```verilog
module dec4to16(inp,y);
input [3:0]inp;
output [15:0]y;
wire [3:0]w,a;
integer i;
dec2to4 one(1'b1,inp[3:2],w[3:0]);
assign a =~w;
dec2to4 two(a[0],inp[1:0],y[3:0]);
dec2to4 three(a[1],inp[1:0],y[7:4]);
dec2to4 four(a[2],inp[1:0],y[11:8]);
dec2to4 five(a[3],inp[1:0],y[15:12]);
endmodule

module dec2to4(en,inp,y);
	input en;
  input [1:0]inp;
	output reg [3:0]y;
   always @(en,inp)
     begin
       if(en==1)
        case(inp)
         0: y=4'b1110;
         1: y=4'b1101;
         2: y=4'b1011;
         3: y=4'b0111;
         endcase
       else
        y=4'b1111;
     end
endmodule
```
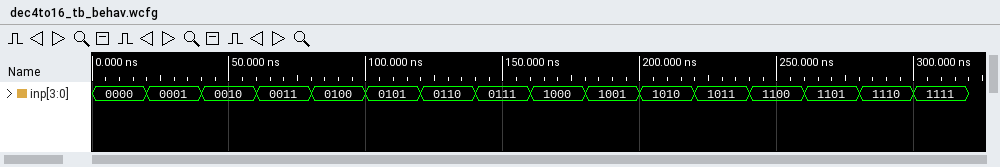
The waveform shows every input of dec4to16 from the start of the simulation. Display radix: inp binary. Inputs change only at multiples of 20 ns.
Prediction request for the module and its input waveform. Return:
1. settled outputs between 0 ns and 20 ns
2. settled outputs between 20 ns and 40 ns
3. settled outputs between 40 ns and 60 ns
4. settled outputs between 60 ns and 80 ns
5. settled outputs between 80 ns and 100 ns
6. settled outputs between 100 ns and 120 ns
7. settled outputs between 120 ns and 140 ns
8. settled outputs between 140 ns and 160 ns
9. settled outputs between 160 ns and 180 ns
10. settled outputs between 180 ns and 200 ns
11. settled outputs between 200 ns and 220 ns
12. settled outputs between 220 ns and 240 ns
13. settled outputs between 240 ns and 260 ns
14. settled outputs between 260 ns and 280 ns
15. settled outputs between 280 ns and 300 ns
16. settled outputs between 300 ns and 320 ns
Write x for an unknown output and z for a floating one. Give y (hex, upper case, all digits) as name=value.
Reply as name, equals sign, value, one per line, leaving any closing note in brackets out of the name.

settled outputs between 0 ns and 20 ns = y=FFFE
settled outputs between 20 ns and 40 ns = y=FFFD
settled outputs between 40 ns and 60 ns = y=FFFB
settled outputs between 60 ns and 80 ns = y=FFF7
settled outputs between 80 ns and 100 ns = y=FFEF
settled outputs between 100 ns and 120 ns = y=FFDF
settled outputs between 120 ns and 140 ns = y=FFBF
settled outputs between 140 ns and 160 ns = y=FF7F
settled outputs between 160 ns and 180 ns = y=FEFF
settled outputs between 180 ns and 200 ns = y=FDFF
settled outputs between 200 ns and 220 ns = y=FBFF
settled outputs between 220 ns and 240 ns = y=F7FF
settled outputs between 240 ns and 260 ns = y=EFFF
settled outputs between 260 ns and 280 ns = y=DFFF
settled outputs between 280 ns and 300 ns = y=BFFF
settled outputs between 300 ns and 320 ns = y=7FFF
